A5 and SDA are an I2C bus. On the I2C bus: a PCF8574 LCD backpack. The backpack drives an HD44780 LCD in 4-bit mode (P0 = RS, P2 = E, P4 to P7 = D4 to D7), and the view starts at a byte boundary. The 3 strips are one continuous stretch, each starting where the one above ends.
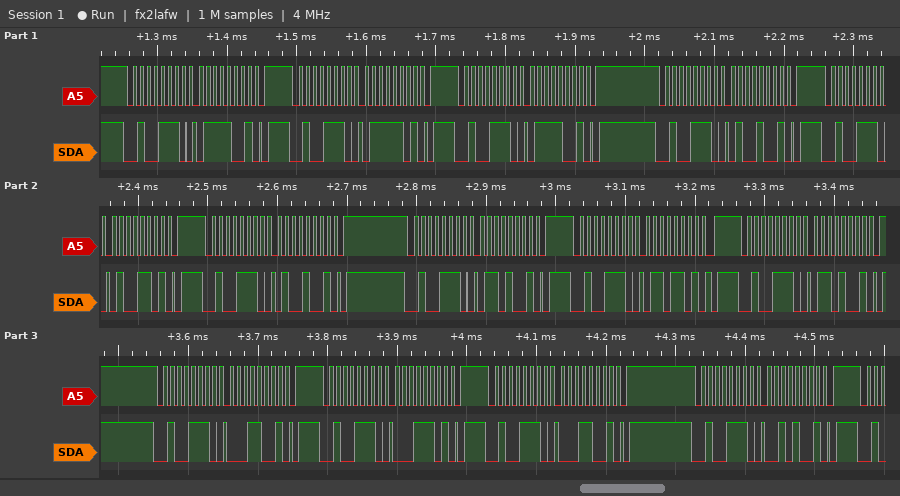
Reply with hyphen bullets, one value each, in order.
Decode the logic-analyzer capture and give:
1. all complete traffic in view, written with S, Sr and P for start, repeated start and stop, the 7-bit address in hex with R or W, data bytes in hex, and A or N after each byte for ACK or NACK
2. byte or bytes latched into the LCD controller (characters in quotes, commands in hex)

- S 27W A 79 A P S 27W A 7D A P S 27W A 79 A P S 27W A 49 A P S 27W A 4D A P S 27W A 49 A P S 27W A 69 A P S 27W A 6D A P S 27W A 69 A P S 27W A 19 A P S 27W A 1D A P S 27W A 19 A P S 27W A 29 A P
- 't' 'a'
